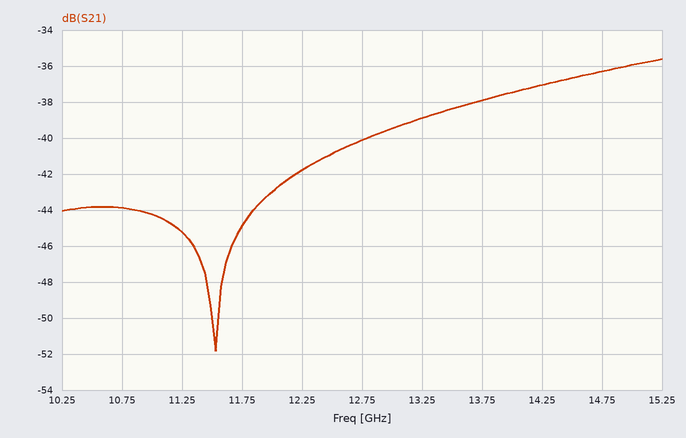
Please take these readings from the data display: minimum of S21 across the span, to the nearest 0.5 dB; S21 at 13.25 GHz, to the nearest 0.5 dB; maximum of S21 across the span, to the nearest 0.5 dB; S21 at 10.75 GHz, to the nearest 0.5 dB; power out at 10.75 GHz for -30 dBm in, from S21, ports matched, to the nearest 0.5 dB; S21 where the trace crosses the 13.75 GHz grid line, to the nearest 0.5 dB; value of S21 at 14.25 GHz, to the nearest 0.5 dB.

-52.0 dB
-39.0 dB
-35.5 dB
-44.0 dB
-74.0 dBm
-38.0 dB
-37.0 dB
